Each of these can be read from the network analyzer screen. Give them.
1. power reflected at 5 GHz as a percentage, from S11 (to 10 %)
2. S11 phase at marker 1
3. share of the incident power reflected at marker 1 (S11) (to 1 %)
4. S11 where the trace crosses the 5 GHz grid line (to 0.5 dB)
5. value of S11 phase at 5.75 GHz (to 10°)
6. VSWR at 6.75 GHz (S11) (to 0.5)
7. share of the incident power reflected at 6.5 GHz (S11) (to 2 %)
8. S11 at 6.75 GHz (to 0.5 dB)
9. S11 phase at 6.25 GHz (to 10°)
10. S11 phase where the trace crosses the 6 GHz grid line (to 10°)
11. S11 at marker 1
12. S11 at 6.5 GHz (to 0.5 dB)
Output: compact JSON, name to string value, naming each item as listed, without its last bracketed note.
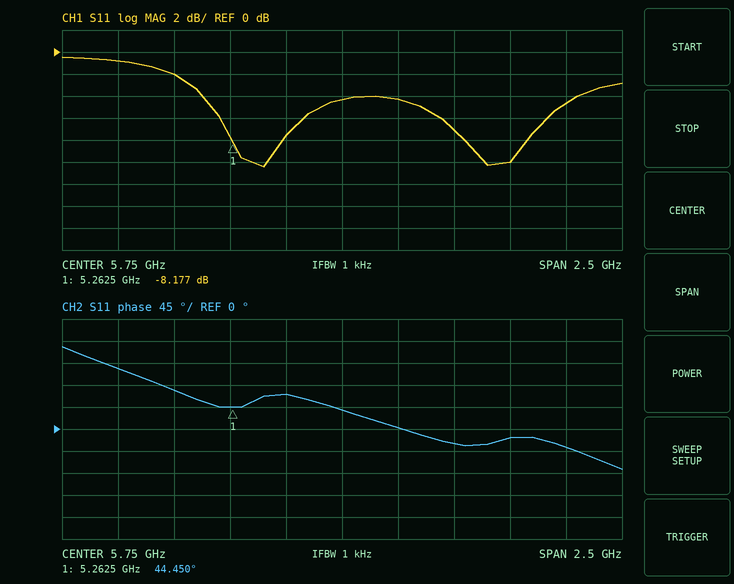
{"power reflected at 5 GHz as a percentage, from S11": "60 %", "S11 phase at marker 1": "44.450°", "share of the incident power reflected at marker 1 (S11)": "15 %", "S11 where the trace crosses the 5 GHz grid line": "-2.0 dB", "value of S11 phase at 5.75 GHz": "40°", "VSWR at 6.75 GHz (S11)": "4.0", "share of the incident power reflected at 6.5 GHz (S11)": "10 %", "S11 at 6.75 GHz": "-4.5 dB", "S11 phase at 6.25 GHz": "-30°", "S11 phase where the trace crosses the 6 GHz grid line": "0°", "S11 at marker 1": "-8.177 dB", "S11 at 6.5 GHz": "-10.0 dB"}
